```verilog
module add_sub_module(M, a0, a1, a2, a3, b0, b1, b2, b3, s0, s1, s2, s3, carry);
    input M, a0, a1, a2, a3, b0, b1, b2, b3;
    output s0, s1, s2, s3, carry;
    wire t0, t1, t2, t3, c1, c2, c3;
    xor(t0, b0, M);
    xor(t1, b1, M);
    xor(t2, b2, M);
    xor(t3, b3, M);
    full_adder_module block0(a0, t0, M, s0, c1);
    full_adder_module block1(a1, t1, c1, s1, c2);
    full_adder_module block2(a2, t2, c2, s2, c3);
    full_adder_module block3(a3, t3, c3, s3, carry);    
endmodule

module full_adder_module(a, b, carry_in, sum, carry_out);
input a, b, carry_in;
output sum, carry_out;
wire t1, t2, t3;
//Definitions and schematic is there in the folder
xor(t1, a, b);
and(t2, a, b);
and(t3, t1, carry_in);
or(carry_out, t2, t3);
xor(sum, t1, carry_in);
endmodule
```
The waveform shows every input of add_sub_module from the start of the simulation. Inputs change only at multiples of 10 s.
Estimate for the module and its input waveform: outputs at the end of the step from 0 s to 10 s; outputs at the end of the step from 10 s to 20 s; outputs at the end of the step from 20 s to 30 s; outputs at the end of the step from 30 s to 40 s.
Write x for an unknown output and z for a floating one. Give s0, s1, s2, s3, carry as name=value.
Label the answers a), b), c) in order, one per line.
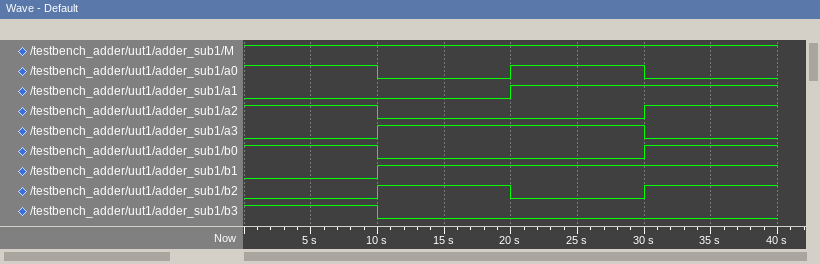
a) s0=0, s1=0, s2=1, s3=1, carry=0
b) s0=0, s1=1, s2=0, s3=0, carry=1
c) s0=1, s1=0, s2=0, s3=1, carry=1
d) s0=1, s1=1, s2=1, s3=1, carry=0
